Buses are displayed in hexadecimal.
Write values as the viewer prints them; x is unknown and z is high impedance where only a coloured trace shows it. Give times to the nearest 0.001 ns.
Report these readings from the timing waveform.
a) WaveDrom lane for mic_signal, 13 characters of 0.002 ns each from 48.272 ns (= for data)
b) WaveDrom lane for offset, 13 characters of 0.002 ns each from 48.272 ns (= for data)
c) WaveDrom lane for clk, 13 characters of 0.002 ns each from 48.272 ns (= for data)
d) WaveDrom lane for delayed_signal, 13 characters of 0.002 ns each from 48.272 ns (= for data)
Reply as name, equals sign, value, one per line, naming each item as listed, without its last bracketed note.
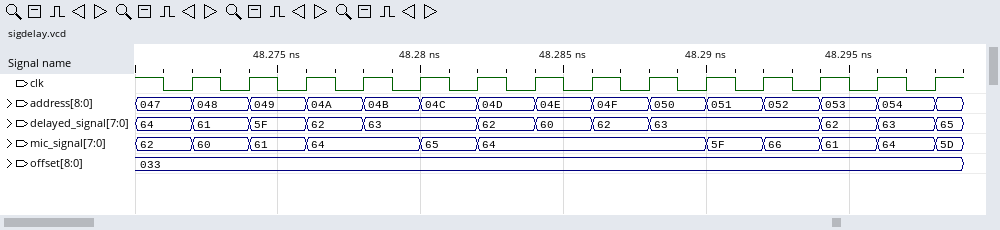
WaveDrom lane for mic_signal, 13 characters of 0.002 ns each from 48.272 ns = {name: 'mic_signal', wave: '===.==...====', data: '60 61 64 65 64 5F 66 61 64'}
WaveDrom lane for offset, 13 characters of 0.002 ns each from 48.272 ns = {name: 'offset', wave: '=............', data: '033'}
WaveDrom lane for clk, 13 characters of 0.002 ns each from 48.272 ns = {name: 'clk', wave: 'p............'}
WaveDrom lane for delayed_signal, 13 characters of 0.002 ns each from 48.272 ns = {name: 'delayed_signal', wave: '====.====..==', data: '61 5F 62 63 62 60 62 63 62 63'}
